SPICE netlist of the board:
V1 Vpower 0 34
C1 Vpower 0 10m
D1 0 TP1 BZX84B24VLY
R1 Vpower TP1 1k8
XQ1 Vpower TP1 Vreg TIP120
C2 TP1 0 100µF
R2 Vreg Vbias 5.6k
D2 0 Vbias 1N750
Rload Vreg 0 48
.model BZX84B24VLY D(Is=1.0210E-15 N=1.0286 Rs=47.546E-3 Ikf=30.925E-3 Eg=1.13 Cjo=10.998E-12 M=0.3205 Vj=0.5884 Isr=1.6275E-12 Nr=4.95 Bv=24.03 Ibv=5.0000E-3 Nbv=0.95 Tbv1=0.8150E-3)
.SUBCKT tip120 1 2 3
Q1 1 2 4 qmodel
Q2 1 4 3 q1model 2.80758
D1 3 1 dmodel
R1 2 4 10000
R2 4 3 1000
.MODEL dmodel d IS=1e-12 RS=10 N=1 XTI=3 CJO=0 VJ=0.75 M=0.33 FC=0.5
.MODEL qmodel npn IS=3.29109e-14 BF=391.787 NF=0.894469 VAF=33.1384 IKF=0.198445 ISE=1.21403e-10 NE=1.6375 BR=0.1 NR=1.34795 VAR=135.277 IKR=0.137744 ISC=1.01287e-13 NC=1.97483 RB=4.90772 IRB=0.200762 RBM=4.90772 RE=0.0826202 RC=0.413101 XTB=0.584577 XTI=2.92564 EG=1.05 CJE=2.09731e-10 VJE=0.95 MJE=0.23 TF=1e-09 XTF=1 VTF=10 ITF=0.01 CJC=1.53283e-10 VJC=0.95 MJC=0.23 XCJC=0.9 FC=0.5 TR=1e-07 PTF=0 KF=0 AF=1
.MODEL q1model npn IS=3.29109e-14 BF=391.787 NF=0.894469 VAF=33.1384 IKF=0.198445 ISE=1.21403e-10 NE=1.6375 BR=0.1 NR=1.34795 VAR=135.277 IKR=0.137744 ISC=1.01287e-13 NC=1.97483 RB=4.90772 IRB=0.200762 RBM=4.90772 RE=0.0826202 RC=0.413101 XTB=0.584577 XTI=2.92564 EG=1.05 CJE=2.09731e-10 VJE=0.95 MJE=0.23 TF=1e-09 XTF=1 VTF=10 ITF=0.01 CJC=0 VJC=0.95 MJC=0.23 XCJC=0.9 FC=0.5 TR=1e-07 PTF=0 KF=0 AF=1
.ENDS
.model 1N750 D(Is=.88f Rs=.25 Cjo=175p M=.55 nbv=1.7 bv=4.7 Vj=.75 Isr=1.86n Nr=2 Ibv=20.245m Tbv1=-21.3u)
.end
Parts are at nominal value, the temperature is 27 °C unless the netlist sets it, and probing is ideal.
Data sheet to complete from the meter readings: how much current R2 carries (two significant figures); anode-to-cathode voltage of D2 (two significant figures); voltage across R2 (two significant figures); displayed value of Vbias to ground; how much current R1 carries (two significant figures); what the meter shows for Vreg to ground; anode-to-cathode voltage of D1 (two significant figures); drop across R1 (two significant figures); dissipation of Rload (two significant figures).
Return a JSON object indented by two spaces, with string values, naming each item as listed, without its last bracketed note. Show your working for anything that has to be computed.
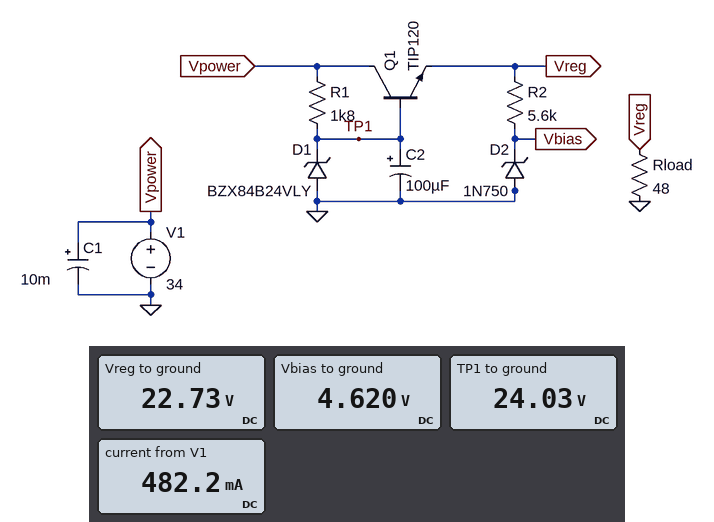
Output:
{
  "how much current R2 carries": "(22.73 V - 4.62 V) / 5.6 kΩ = 3.2 mA",
  "anode-to-cathode voltage of D2": "0 V - 4.62 V = -4.6 V",
  "voltage across R2": "22.73 V - 4.62 V = 18 V",
  "displayed value of Vbias to ground": "4.620 V",
  "how much current R1 carries": "(34 V - 24.03 V) / 1.8 kΩ = 5.5 mA",
  "what the meter shows for Vreg to ground": "22.73 V",
  "anode-to-cathode voltage of D1": "0 V - 24.03 V = -24 V",
  "drop across R1": "34 V - 24.03 V = 10 V",
  "dissipation of Rload": "(22.73 V)^2 / 48 Ω = 11 W"
}
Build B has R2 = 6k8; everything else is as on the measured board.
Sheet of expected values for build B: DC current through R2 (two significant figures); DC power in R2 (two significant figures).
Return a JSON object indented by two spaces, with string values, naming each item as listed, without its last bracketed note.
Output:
{
  "DC current through R2": "2.7 mA",
  "DC power in R2": "48 mW"
}
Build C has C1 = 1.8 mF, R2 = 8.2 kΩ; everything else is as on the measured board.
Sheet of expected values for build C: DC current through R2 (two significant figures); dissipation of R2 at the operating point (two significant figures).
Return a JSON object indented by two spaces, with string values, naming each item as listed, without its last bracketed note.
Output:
{
  "DC current through R2": "2.2 mA",
  "dissipation of R2 at the operating point": "40 mW"
}
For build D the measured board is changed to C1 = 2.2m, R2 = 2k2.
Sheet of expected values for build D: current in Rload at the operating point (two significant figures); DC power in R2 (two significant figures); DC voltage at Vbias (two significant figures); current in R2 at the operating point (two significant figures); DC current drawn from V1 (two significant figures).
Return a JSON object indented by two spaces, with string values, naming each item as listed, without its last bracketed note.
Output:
{
  "current in Rload at the operating point": "470 mA",
  "DC power in R2": "150 mW",
  "DC voltage at Vbias": "4.7 V",
  "current in R2 at the operating point": "8.2 mA",
  "DC current drawn from V1": "490 mA"
}
